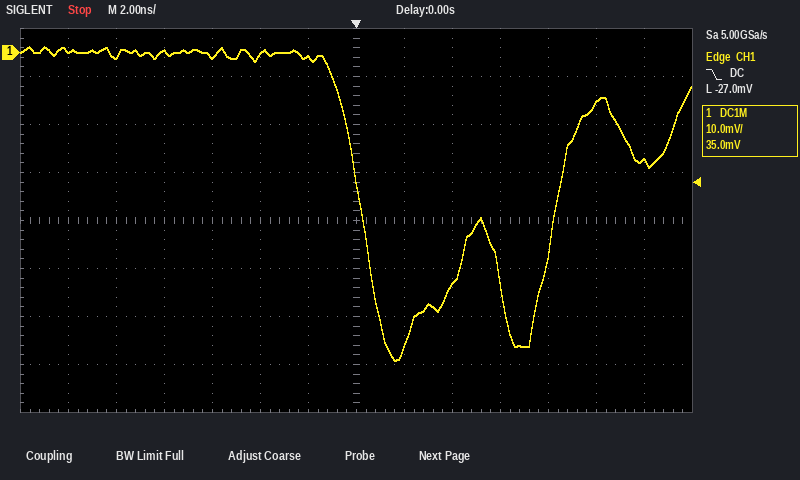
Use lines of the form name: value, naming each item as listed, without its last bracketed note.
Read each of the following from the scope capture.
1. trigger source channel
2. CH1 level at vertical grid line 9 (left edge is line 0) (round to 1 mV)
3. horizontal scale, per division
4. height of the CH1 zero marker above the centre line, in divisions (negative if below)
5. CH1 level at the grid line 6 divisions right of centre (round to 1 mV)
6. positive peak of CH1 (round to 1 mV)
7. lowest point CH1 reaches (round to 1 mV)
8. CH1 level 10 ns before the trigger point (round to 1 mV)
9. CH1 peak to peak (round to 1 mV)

trigger source channel: CH1
CH1 level at vertical grid line 9 (left edge is line 0): -48 mV
horizontal scale, per division: 2 ns
height of the CH1 zero marker above the centre line, in divisions: +3.5 div
CH1 level at the grid line 6 divisions right of centre: -22 mV
positive peak of CH1: 1 mV
lowest point CH1 reaches: -64 mV
CH1 level 10 ns before the trigger point: -1 mV
CH1 peak to peak: 65 mV
